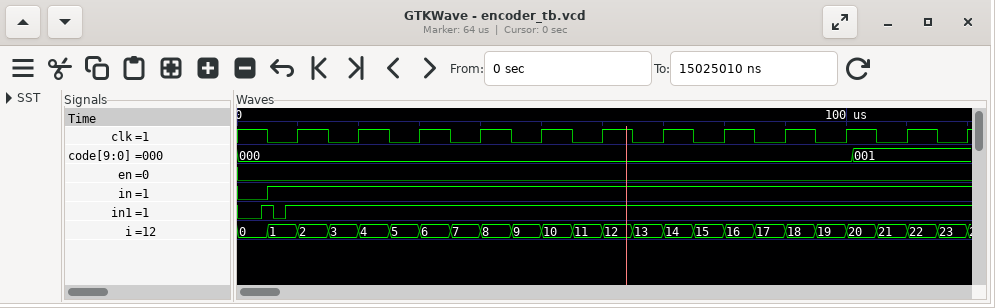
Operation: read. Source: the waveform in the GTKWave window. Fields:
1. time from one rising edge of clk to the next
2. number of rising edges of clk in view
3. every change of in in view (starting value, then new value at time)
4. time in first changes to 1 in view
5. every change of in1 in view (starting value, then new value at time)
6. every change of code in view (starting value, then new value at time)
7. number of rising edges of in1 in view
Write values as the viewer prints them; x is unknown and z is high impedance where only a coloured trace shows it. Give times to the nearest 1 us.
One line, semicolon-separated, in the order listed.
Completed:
10 us; 12; 0, 1 at 5 us; 5 us; 0, 1 at 4 us, 0 at 6 us, 1 at 8 us; 000, 001 at 101 us; 2
